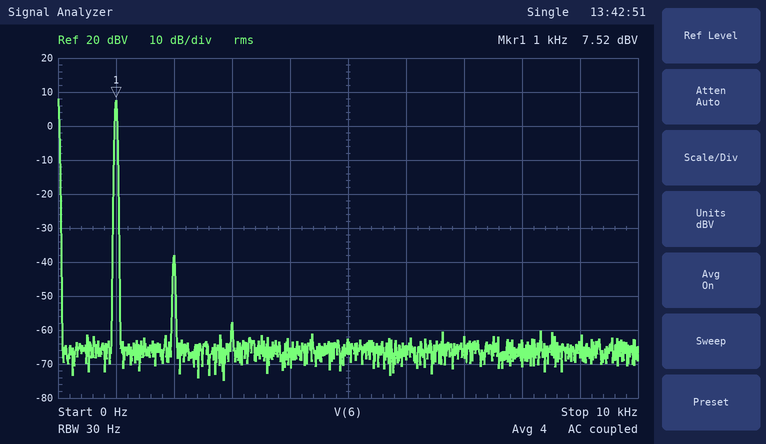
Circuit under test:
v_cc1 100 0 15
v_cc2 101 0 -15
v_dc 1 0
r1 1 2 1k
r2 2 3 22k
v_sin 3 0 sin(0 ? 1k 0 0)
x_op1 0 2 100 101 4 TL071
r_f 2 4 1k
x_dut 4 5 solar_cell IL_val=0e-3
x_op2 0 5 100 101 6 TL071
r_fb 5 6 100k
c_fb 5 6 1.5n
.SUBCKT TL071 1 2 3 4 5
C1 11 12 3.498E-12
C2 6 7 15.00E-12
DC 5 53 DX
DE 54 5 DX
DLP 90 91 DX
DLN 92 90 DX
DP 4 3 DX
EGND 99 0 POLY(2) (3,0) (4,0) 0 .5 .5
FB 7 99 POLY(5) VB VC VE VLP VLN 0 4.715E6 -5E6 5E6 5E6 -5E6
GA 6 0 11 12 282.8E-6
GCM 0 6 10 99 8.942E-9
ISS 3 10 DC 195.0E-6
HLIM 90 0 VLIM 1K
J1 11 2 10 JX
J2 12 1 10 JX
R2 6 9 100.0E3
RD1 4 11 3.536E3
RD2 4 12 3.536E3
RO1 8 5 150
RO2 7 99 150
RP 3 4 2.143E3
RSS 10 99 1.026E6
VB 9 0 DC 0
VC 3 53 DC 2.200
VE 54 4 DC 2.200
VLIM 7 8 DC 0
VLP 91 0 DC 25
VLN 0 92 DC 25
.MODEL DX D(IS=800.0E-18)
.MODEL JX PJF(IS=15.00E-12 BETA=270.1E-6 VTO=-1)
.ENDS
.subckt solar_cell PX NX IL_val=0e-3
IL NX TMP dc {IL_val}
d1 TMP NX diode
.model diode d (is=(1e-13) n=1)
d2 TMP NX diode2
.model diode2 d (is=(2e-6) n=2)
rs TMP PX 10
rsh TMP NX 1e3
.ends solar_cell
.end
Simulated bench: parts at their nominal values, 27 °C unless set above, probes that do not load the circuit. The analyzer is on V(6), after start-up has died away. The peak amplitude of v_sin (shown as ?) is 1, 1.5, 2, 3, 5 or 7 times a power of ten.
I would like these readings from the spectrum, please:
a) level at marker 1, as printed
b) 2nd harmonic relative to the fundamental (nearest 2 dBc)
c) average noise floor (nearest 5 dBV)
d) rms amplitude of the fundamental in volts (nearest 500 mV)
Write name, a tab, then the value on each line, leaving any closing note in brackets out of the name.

level at marker 1, as printed	7.52 dBV
2nd harmonic relative to the fundamental	-46 dBc
average noise floor	-65 dBV
rms amplitude of the fundamental in volts	2.5 V
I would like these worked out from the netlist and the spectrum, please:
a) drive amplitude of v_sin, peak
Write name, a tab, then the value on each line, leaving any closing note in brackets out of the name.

drive amplitude of v_sin, peak	1 V
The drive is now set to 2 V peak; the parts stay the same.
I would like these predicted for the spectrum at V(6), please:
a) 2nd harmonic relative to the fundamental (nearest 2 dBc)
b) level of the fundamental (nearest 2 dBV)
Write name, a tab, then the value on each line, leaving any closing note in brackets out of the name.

2nd harmonic relative to the fundamental	-38 dBc
level of the fundamental	14 dBV
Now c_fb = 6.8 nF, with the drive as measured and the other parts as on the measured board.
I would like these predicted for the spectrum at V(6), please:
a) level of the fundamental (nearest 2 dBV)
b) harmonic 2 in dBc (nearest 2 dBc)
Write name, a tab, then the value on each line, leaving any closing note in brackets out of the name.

level of the fundamental	-2 dBV
harmonic 2 in dBc	-48 dBc
